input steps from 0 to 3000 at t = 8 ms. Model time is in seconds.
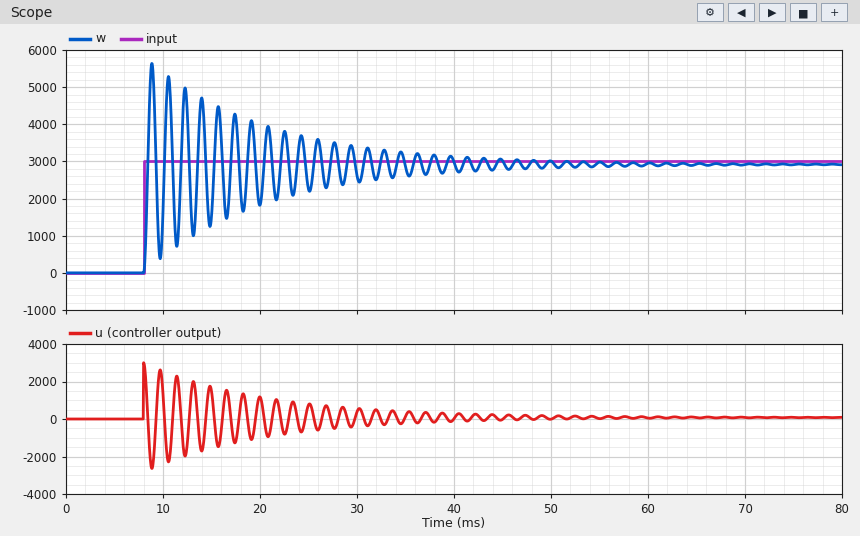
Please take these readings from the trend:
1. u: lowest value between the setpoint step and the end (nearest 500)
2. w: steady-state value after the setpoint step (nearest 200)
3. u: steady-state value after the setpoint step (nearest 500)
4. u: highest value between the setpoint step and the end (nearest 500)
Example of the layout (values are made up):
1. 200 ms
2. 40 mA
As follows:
1. -2500
2. 3000
3. 0
4. 3000
